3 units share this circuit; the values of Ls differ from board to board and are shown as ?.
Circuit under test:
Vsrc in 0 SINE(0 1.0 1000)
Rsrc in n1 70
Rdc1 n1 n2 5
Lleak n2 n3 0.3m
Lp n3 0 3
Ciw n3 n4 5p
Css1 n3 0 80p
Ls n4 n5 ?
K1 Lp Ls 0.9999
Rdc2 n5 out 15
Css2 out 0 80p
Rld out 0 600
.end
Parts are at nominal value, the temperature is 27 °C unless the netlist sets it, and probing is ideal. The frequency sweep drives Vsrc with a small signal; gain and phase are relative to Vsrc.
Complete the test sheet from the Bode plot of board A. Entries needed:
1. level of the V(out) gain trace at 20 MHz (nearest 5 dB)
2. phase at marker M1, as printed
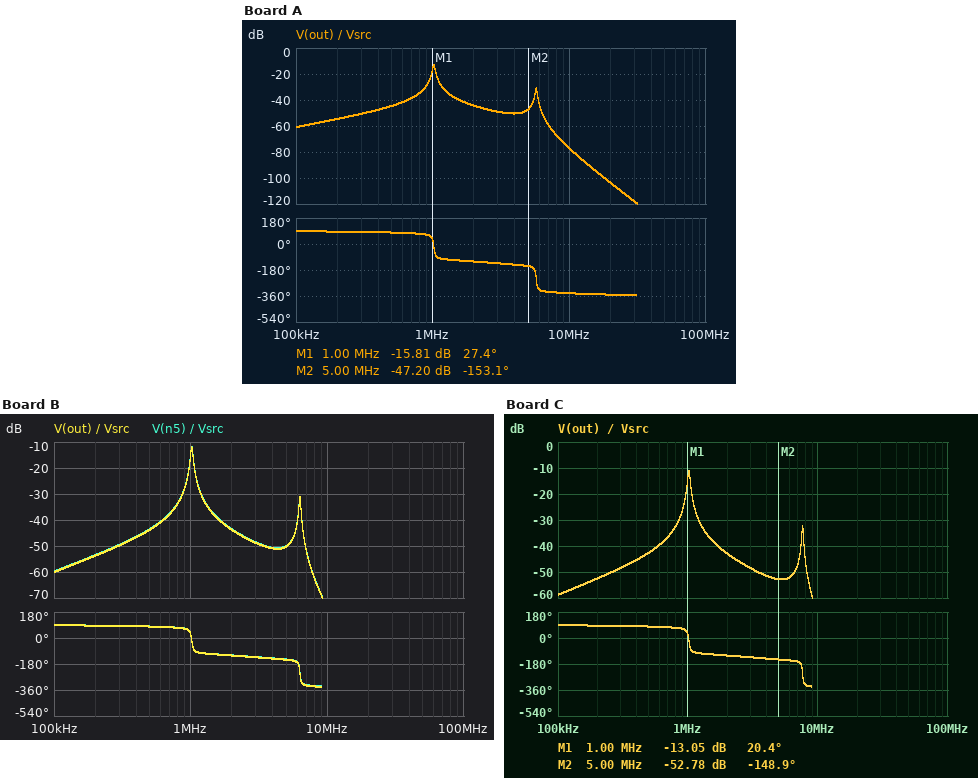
-105 dB
27.4 deg
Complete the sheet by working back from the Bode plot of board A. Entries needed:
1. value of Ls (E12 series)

820 mH
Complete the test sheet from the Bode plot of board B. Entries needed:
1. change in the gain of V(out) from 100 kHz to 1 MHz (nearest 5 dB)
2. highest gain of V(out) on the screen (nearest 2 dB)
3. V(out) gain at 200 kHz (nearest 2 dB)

45 dB
-12 dB
-54 dB
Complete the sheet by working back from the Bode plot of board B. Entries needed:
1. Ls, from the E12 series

680 mH
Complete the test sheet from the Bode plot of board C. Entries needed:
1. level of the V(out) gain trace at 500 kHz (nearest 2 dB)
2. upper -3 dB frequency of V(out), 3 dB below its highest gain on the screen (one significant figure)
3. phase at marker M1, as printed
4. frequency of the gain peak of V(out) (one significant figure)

-42 dB
1 MHz
20.4 deg
1 MHz
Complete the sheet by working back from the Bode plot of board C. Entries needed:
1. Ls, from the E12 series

470 mH
